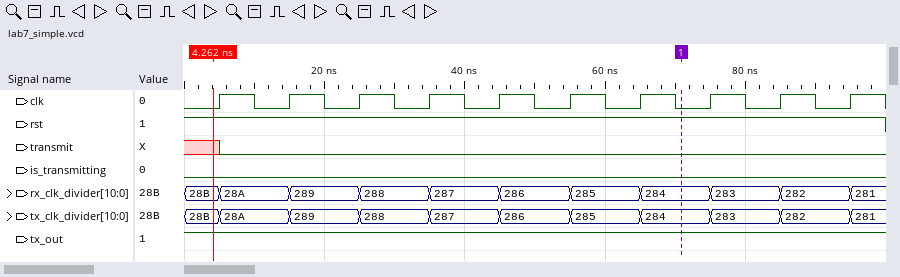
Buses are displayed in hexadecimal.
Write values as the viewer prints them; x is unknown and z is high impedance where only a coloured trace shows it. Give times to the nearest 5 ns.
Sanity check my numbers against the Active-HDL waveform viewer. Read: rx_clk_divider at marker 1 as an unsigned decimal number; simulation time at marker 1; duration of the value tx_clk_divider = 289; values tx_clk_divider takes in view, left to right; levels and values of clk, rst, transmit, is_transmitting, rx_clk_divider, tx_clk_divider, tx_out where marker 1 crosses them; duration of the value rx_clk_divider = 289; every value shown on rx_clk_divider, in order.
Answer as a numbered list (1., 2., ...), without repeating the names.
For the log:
1. 644
2. 70 ns
3. 10 ns
4. 28B, 28A, 289, 288, 287, 286, 285, 284, 283, 282, 281
5. clk=0, rst=1, transmit=0, is_transmitting=0, rx_clk_divider=284, tx_clk_divider=284, tx_out=1
6. 10 ns
7. 28B, 28A, 289, 288, 287, 286, 285, 284, 283, 282, 281
